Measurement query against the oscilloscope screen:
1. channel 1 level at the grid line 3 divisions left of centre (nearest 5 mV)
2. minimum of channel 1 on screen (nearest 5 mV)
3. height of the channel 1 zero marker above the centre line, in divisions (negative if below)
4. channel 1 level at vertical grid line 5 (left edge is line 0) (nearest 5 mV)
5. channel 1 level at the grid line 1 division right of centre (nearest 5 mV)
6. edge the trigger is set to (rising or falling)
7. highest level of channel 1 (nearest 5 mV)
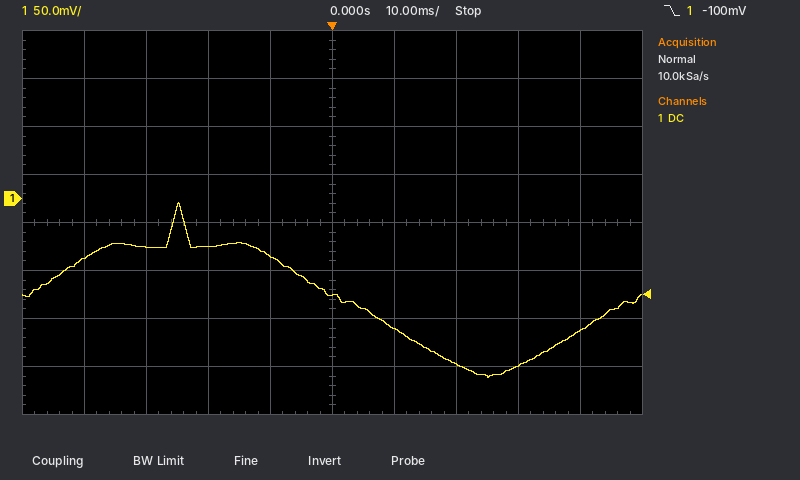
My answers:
-50 mV
-185 mV
+0.5 div
-100 mV
-135 mV
falling
-5 mV
